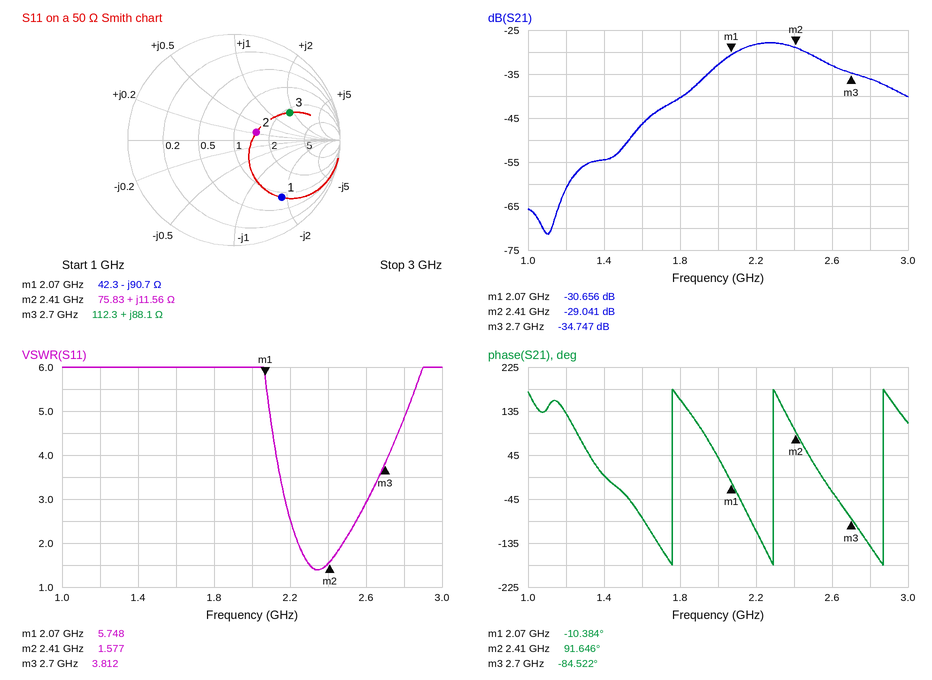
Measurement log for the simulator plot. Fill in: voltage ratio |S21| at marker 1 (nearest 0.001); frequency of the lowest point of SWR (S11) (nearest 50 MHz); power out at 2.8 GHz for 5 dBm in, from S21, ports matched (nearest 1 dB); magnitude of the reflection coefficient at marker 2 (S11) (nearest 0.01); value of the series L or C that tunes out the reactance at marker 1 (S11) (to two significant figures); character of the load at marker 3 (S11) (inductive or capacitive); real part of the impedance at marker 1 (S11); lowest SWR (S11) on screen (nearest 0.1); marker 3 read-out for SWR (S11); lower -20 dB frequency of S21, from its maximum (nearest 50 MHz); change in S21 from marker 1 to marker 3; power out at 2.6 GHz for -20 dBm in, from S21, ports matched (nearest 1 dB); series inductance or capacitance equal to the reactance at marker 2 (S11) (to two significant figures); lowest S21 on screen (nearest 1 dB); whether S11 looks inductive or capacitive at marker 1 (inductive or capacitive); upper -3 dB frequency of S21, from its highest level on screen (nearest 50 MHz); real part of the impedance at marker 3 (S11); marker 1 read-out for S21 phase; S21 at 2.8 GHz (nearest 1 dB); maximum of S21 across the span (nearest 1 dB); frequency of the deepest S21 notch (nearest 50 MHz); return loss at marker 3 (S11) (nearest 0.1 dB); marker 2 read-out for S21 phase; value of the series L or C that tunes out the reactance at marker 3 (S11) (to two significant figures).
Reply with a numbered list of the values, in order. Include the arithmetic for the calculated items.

1. 10^(-30.656/20) ≈ 0.029
2. 2.35 GHz
3. 5 dBm + (-36 dB) = -31 dBm
4. 0.22
5. L = 90.7 Ω/(2π × 2.07 GHz) ≈ 7.0 nH
6. inductive
7. 42.3 Ω
8. 1.4
9. 3.812
10. 1.55 GHz
11. -34.747 − (-30.656) = -4.091 dB
12. -20 dBm + (-33 dB) = -53 dBm
13. L = 11.56 Ω/(2π × 2.41 GHz) ≈ 763 pH, so 760 pH to two significant figures
14. -71 dB
15. capacitive
16. 2.50 GHz
17. 112.3 Ω
18. -10.384°
19. -36 dB
20. -28 dB
21. 1.10 GHz
22. 4.7 dB
23. 91.646°
24. C = 1/(2π × 2.7 GHz × 88.1 Ω) ≈ 669 fF, so 670 fF to two significant figures
